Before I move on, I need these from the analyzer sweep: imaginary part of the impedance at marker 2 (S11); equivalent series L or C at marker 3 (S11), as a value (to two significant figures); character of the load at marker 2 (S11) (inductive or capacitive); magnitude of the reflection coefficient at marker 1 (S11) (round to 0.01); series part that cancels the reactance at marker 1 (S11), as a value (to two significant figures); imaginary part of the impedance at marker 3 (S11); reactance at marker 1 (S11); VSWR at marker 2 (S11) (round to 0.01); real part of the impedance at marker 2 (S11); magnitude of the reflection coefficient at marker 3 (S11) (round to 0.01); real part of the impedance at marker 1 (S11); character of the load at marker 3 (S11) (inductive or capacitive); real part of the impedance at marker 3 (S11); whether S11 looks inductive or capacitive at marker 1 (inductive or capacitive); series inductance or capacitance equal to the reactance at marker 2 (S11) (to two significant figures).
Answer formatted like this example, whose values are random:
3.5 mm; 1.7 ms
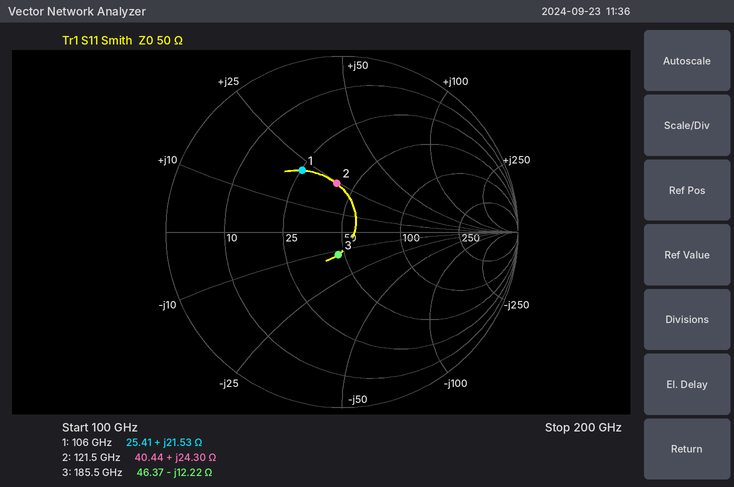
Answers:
+24.30 Ω; 70 fF; inductive; 0.42; 70 fF; -12.22 Ω; +21.53 Ω; 1.77; 40.44 Ω; 0.13; 25.41 Ω; capacitive; 46.37 Ω; inductive; 32 pH
